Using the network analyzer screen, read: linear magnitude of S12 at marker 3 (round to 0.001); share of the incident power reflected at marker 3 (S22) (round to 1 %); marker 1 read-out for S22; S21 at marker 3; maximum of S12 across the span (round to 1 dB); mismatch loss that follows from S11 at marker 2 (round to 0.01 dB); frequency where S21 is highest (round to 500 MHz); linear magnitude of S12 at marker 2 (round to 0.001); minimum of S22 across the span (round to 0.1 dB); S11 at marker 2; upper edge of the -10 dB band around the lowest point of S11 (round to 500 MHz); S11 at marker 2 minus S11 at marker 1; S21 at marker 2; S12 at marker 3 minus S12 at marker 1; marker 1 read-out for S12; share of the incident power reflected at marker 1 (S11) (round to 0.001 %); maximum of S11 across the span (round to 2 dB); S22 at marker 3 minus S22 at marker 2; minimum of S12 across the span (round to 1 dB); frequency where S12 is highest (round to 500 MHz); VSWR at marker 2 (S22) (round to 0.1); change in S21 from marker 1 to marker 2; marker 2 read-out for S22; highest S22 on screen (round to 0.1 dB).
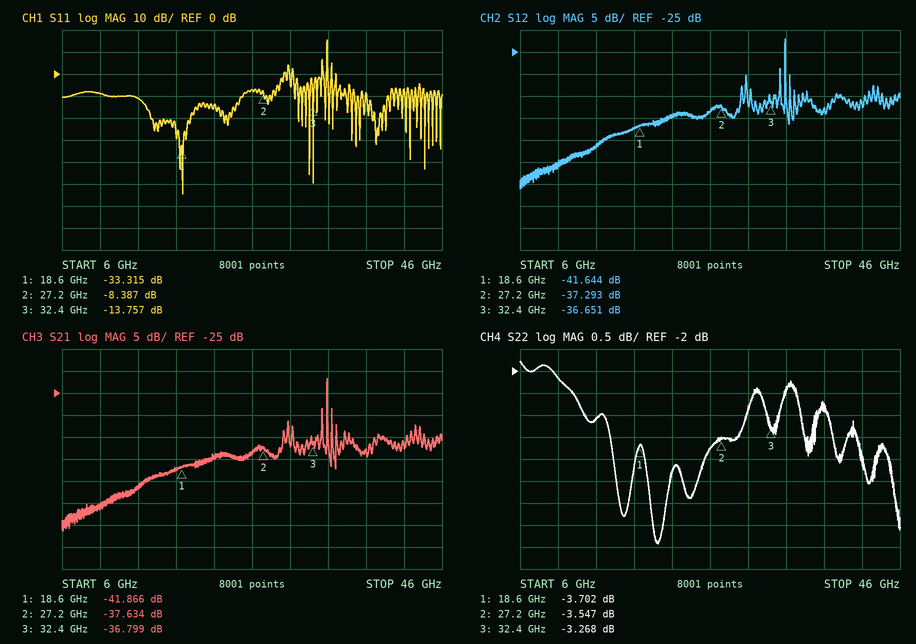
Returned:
0.015
47 %
-3.702 dB
-36.799 dB
-22 dB
0.68 dB
34.0 GHz
0.014
-5.9 dB
-8.387 dB
25.0 GHz
24.928 dB
-37.634 dB
4.993 dB
-41.644 dB
0.047 %
16 dB
0.279 dB
-56 dB
34.0 GHz
5.0
4.232 dB
-3.547 dB
-1.8 dB
